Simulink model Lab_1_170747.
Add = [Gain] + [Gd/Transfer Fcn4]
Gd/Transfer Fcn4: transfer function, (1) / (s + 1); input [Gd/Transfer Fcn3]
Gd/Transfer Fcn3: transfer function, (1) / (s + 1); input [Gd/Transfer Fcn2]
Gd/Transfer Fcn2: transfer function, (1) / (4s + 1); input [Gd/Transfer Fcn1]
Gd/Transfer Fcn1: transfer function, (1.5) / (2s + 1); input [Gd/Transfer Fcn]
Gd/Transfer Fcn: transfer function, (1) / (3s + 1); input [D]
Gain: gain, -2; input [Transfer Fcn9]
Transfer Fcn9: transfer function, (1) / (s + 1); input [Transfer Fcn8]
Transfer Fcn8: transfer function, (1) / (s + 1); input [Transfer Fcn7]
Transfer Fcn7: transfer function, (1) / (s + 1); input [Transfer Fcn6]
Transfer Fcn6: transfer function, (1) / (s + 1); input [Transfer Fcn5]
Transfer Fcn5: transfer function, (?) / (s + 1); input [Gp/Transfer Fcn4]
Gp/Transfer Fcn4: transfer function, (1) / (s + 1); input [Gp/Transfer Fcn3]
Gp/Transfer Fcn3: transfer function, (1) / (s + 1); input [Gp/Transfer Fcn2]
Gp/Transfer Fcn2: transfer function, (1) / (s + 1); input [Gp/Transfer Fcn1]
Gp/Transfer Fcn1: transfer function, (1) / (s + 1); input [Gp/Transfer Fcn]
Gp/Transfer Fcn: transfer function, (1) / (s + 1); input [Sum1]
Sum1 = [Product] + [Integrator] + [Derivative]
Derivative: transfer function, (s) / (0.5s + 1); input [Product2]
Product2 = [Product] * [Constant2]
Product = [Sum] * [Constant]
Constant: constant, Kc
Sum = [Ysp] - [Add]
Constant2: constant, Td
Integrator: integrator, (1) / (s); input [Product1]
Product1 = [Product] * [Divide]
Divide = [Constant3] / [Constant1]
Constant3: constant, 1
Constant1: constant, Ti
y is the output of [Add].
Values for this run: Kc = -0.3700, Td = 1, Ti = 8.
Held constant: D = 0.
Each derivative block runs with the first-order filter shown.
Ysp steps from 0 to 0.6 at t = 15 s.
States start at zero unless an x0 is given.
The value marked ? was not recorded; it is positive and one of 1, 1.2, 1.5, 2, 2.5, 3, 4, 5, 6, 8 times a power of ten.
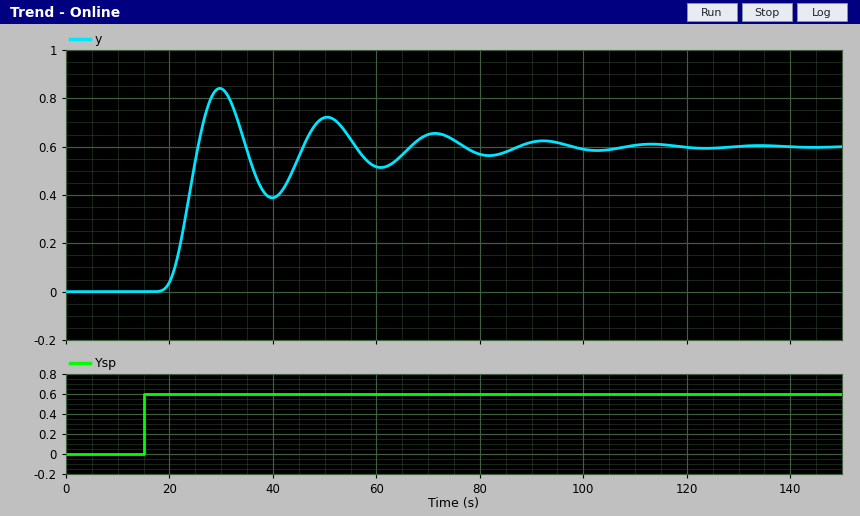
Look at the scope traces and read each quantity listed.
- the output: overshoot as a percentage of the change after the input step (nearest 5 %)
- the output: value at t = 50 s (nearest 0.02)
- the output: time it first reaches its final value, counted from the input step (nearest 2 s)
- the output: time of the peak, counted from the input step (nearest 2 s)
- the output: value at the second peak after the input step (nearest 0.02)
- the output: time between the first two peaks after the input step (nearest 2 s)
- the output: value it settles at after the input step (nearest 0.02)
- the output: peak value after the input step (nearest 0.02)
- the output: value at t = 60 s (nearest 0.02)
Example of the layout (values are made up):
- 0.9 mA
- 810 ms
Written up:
- 40 %
- 0.72
- 10 s
- 14 s
- 0.72
- 20 s
- 0.60
- 0.84
- 0.52
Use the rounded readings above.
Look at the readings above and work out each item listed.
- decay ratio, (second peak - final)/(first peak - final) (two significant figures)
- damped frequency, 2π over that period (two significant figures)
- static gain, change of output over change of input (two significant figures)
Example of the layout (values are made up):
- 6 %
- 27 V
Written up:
- 0.50
- 0.31 rad/s
- 1.0
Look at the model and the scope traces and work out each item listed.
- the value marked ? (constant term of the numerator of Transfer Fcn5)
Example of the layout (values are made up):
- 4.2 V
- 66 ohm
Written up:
- 1.5
